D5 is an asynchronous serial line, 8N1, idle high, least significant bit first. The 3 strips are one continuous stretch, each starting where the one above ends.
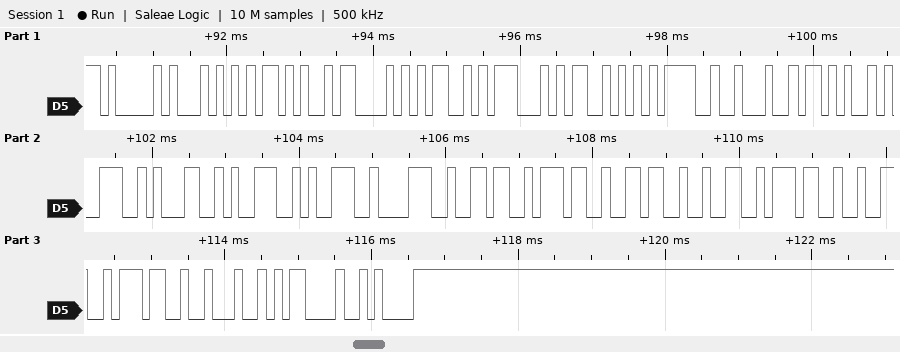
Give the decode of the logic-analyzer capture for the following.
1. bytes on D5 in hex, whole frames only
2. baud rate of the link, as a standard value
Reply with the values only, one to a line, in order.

41 54 2B 43 4D 47 53 3D 22 2B 39 31 39 39 38 36 37 36 32 37 32 37 22 0D 0A
9600 baud
